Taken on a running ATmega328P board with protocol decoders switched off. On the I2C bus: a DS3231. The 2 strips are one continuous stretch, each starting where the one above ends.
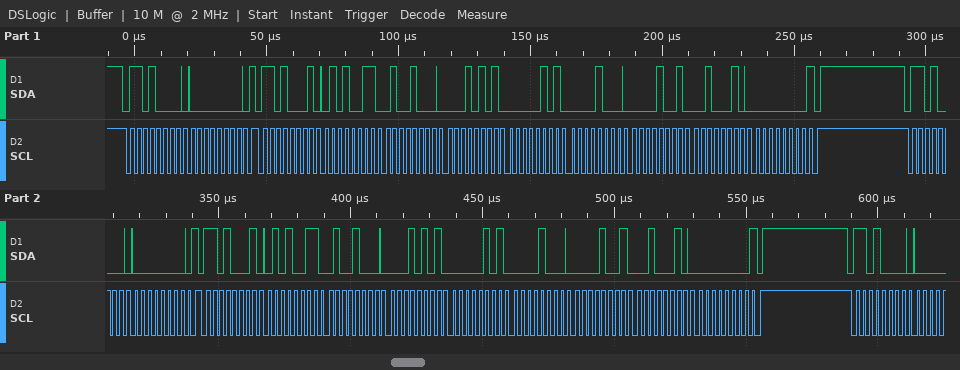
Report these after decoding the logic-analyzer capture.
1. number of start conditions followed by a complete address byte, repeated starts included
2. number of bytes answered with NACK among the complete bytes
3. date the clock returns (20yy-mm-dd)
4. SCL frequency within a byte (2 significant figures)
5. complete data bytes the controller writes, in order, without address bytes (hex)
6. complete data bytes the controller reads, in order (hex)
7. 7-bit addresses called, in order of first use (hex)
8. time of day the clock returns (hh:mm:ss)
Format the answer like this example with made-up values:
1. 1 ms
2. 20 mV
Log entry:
1. 5
2. 2
3. 2022-09-08
4. 400 kHz
5. 00 00
6. 53 48 15 05 08 09 22 00 53 48 15 05 08 09 22 00
7. 0x68
8. 15:48:53
